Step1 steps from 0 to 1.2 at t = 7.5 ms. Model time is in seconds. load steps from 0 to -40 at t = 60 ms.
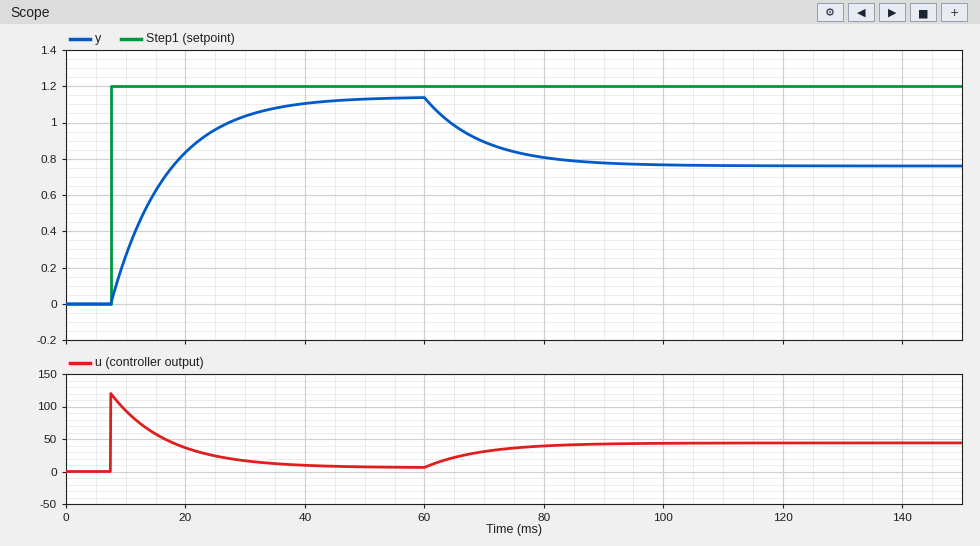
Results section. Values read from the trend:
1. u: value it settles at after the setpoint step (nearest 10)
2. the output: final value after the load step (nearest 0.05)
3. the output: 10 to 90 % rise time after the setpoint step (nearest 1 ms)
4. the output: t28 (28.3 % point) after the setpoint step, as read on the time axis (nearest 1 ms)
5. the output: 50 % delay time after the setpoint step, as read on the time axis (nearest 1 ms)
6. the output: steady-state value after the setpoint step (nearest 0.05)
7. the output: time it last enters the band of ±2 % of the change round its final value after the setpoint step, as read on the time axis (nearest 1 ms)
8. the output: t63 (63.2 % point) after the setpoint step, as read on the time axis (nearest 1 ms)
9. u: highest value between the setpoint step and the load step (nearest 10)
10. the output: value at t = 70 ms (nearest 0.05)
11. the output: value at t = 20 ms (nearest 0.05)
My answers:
10
0.75
20 ms
11 ms
14 ms
1.15
42 ms
17 ms
120
0.90
0.85
